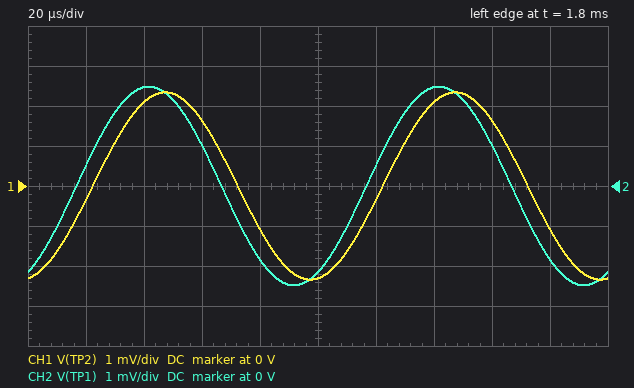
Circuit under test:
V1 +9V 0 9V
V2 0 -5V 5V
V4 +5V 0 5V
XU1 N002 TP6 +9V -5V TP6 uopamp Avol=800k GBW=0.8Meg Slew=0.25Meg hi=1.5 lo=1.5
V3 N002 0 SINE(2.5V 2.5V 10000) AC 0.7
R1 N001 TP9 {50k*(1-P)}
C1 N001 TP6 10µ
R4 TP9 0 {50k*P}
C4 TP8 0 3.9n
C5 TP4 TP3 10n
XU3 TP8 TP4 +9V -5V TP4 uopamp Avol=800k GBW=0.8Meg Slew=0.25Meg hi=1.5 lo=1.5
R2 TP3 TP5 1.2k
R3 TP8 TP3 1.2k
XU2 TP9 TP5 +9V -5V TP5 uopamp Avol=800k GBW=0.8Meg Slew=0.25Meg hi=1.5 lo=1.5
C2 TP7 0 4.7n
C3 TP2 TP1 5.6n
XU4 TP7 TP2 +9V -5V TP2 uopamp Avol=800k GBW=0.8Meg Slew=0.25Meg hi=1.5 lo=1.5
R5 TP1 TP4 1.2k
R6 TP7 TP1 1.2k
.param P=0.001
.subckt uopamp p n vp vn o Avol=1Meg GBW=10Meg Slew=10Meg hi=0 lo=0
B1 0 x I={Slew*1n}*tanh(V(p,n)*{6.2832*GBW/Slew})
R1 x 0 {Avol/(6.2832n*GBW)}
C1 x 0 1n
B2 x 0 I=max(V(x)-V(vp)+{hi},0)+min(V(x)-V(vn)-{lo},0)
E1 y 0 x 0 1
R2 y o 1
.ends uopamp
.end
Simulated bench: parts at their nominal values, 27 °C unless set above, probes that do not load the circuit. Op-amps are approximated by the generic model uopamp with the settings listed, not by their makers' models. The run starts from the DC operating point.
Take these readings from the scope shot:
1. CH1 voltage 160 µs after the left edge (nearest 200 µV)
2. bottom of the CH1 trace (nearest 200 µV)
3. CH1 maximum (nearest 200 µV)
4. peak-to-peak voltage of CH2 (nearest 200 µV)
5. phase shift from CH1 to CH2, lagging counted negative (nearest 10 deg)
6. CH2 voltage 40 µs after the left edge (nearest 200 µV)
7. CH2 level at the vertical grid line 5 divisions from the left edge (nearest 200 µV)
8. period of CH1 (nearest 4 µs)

1.6 mV
-2.4 mV
2.4 mV
5.0 mV
20 deg
2.4 mV
-2.2 mV
100 µs
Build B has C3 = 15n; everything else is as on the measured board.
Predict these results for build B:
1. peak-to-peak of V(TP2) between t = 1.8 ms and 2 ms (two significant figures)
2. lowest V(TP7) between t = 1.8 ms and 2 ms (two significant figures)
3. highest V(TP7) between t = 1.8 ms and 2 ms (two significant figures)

5.6 mV
-2.8 mV
2.8 mV
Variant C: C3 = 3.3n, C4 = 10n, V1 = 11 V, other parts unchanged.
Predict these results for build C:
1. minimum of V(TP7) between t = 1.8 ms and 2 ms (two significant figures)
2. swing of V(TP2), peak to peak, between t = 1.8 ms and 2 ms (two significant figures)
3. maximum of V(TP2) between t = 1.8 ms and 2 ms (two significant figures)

-1.4 mV
2.8 mV
1.4 mV
